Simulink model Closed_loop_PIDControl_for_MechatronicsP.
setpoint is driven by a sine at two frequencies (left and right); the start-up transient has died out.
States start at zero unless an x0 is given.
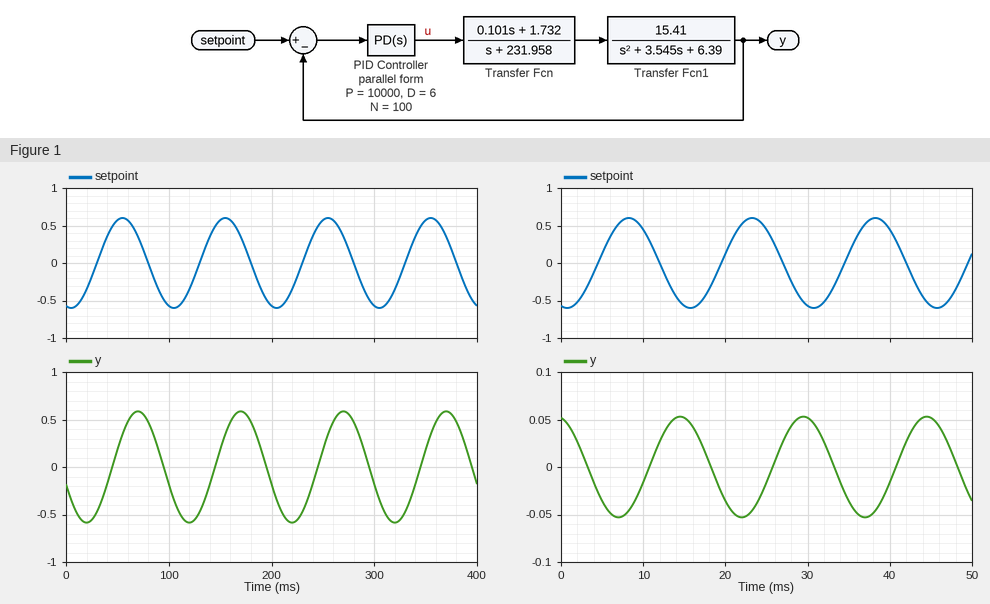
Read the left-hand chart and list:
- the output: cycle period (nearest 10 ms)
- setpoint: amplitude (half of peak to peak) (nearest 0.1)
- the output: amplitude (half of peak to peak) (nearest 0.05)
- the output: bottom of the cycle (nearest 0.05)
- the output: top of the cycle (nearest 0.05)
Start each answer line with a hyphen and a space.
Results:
- 100 ms
- 0.6
- 0.60
- -0.60
- 0.60
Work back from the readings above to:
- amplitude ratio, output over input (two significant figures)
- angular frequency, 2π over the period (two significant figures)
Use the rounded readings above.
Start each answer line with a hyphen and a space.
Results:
- 1.0
- 0.063 rad/ms
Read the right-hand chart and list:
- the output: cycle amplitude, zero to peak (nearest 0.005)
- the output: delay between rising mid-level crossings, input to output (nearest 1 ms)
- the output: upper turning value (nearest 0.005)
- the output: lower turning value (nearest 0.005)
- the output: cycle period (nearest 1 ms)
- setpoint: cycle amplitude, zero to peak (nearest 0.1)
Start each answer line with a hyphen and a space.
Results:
- 0.055
- 6 ms
- 0.055
- -0.055
- 15 ms
- 0.6
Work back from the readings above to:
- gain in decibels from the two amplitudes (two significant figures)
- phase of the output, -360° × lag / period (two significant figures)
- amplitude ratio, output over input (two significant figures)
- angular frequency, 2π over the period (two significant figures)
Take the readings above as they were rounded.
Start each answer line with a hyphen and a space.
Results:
- -21 dB
- -140°
- 0.092
- 0.42 rad/ms
